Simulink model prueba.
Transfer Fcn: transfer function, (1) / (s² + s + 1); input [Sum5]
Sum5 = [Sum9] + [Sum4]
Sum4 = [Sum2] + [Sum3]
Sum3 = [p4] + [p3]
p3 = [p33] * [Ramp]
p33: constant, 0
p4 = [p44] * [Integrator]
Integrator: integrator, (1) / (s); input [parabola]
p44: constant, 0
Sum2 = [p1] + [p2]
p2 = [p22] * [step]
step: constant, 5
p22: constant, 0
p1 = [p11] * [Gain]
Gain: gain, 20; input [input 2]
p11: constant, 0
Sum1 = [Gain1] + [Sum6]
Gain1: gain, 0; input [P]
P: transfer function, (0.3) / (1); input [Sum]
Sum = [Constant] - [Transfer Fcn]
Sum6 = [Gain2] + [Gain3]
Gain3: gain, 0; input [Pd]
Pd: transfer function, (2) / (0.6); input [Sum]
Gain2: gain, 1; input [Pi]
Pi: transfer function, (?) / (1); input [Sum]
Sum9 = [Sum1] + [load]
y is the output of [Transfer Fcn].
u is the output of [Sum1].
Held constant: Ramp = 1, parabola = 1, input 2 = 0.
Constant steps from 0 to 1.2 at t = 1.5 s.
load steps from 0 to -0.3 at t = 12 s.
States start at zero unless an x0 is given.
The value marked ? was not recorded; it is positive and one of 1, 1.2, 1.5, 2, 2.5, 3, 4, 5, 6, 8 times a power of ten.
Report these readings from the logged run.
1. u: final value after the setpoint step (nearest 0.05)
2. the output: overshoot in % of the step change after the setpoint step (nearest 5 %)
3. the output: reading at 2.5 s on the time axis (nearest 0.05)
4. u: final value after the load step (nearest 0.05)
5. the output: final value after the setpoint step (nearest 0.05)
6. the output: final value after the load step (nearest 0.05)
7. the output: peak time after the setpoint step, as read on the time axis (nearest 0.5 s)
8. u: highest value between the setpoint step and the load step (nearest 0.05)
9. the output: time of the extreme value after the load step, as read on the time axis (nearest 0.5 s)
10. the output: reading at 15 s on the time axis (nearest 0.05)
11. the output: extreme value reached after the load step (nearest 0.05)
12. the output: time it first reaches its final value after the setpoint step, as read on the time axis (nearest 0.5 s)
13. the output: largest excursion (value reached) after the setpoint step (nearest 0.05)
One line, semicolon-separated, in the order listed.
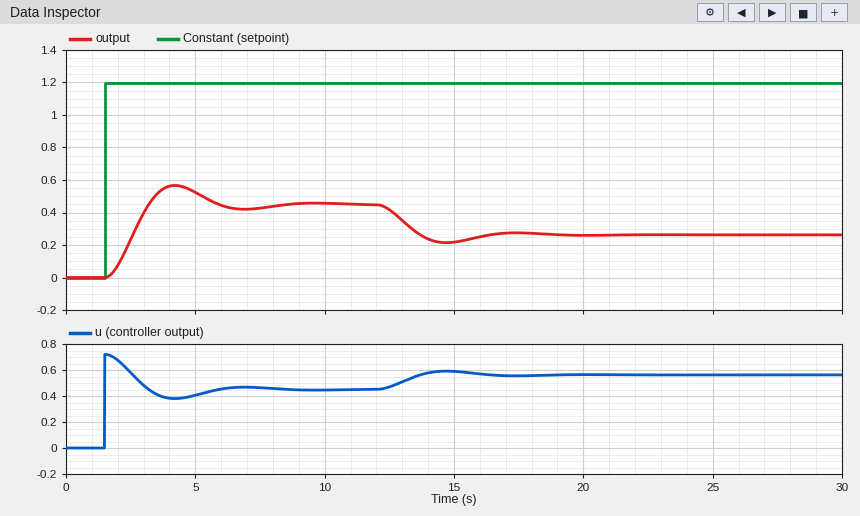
0.45; 25 %; 0.25; 0.55; 0.45; 0.25; 4.0 s; 0.70; 14.5 s; 0.20; 0.20; 3.0 s; 0.55
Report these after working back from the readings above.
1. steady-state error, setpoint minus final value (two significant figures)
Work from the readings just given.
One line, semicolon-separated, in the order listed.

0.75
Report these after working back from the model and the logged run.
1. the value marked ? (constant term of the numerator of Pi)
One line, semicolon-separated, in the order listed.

0.6
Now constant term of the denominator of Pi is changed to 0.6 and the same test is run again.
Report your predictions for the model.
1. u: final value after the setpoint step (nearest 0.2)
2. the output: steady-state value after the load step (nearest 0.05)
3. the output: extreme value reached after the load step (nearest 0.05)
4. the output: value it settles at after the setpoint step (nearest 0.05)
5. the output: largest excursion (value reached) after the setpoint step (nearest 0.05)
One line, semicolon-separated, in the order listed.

0.6; 0.45; 0.40; 0.60; 0.80
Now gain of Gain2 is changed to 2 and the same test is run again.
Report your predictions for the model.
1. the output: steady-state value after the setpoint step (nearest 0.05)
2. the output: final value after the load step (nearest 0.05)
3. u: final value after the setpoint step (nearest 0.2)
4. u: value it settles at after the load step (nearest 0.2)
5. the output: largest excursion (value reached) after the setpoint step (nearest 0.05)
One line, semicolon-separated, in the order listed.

0.65; 0.50; 0.6; 0.8; 0.85
